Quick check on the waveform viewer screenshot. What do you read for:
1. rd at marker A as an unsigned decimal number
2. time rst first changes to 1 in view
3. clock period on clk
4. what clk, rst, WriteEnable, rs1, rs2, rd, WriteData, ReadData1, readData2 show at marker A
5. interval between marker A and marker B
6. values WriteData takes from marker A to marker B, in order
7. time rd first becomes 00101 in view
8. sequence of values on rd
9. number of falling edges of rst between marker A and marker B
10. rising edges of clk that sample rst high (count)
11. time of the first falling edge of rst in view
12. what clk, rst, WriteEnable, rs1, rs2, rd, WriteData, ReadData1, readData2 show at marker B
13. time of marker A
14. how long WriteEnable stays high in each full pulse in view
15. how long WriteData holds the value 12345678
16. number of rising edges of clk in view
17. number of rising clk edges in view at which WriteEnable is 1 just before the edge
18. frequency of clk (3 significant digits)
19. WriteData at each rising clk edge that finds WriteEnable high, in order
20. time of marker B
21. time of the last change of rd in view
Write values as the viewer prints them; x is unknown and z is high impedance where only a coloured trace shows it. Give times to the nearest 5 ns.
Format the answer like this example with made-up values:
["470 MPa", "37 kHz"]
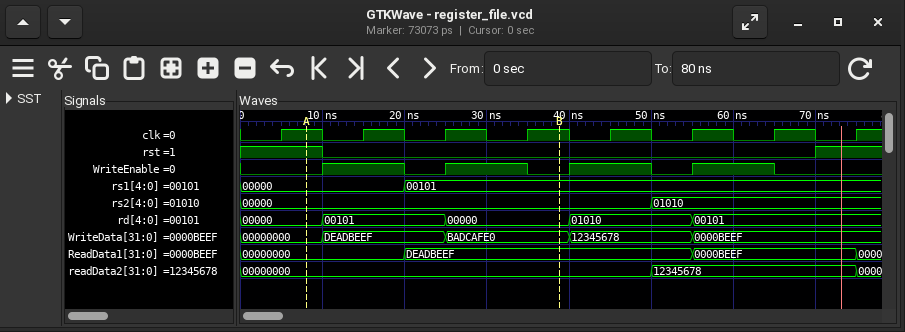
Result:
["0", "70 ns", "10 ns", "clk=1, rst=1, WriteEnable=0, rs1=00000, rs2=00000, rd=00000, WriteData=00000000, ReadData1=00000000, readData2=00000000", "30 ns", "00000000, DEADBEEF, BADCAFE0", "10 ns", "00000, 00101, 00000, 01010, 00101", "1", "2", "10 ns", "clk=1, rst=0, WriteEnable=0, rs1=00101, rs2=00000, rd=00000, WriteData=BADCAFE0, ReadData1=DEADBEEF, readData2=00000000", "10 ns", "10 ns, 10 ns, 10 ns, 10 ns", "15 ns", "8", "4", "100 MHz", "DEADBEEF, BADCAFE0, 12345678, 0000BEEF", "40 ns", "55 ns"]
